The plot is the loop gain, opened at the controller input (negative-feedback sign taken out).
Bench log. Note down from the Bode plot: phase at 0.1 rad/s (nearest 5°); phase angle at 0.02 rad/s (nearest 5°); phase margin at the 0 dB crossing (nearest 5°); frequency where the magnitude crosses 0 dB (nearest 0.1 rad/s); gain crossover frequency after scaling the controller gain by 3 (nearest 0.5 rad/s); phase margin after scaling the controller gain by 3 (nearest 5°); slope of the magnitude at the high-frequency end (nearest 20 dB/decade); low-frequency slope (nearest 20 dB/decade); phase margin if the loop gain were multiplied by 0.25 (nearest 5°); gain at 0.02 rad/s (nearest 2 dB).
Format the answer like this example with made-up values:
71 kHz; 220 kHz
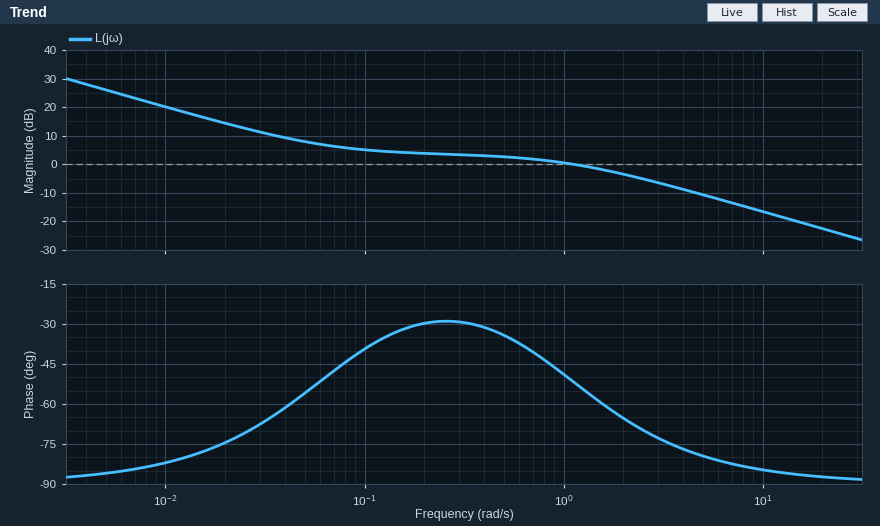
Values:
-40°; -75°; 130°; 1.1 rad/s; 4.5 rad/s; 100°; -20 dB/decade; -20 dB/decade; 110°; 14 dB
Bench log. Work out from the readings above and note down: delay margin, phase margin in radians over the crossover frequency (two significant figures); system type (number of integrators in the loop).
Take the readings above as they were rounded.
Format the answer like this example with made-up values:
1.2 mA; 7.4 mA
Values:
2.1 s; 1
